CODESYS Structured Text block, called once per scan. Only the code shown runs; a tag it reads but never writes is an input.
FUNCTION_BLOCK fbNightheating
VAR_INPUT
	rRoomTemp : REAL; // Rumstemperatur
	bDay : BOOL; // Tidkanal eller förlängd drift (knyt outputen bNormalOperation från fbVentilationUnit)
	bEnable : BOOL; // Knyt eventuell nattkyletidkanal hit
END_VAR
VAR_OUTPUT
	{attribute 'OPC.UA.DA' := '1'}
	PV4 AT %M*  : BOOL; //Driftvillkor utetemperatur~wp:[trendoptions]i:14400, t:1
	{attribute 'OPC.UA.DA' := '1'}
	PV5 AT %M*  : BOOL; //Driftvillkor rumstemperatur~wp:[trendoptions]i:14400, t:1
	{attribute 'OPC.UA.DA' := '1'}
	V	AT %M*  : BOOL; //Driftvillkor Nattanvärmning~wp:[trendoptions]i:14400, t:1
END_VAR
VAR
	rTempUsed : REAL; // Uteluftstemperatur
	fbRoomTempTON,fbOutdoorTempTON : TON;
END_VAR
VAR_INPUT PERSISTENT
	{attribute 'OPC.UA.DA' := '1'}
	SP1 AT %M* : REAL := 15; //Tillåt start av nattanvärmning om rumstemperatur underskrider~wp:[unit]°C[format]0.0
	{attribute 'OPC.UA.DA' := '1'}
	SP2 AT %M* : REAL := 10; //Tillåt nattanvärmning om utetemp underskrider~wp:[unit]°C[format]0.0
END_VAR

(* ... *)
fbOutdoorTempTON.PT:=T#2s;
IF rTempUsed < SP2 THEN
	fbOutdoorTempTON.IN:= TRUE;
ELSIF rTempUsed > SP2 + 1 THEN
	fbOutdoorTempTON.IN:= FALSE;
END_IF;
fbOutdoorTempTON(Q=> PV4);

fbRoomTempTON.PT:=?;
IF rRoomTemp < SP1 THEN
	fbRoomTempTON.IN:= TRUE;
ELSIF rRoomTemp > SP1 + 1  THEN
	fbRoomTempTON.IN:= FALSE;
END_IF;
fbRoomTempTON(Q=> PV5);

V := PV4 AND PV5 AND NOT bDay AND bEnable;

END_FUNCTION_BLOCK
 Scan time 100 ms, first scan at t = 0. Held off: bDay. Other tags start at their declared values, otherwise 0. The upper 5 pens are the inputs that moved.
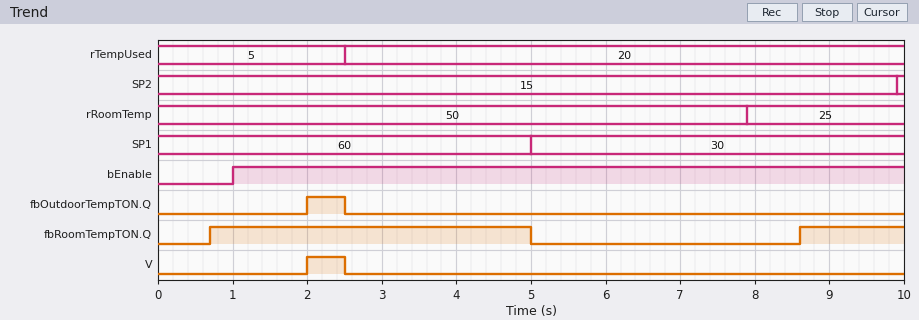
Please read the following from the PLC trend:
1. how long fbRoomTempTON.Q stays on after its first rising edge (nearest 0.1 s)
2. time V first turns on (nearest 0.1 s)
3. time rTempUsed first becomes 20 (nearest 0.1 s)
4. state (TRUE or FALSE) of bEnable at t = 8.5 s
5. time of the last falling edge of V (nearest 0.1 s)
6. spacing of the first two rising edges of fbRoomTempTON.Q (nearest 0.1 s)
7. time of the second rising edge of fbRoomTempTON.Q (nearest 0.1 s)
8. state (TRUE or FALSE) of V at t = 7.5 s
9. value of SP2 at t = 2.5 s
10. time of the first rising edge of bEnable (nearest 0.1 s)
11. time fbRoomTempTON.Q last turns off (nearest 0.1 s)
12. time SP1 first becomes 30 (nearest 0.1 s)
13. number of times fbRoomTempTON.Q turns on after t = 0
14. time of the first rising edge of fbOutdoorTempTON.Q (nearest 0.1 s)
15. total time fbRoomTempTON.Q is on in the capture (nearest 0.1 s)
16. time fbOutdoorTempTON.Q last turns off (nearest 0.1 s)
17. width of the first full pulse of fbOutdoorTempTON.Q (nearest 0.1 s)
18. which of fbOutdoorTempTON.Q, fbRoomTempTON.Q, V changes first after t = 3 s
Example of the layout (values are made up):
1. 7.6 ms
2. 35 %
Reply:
1. 4.3 s
2. 2.0 s
3. 2.5 s
4. TRUE
5. 2.5 s
6. 7.9 s
7. 8.6 s
8. FALSE
9. 15
10. 1.0 s
11. 5.0 s
12. 5.0 s
13. 2
14. 2.0 s
15. 5.7 s
16. 2.5 s
17. 0.5 s
18. fbRoomTempTON.Q
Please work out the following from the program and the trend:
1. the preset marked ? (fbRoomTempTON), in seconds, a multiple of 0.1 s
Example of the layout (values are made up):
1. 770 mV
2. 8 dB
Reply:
1. 0.7 s
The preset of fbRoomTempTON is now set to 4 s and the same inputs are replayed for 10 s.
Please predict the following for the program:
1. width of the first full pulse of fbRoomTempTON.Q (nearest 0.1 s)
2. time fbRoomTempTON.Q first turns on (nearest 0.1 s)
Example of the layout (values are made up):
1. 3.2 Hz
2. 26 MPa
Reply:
1. 1.0 s
2. 4.0 s
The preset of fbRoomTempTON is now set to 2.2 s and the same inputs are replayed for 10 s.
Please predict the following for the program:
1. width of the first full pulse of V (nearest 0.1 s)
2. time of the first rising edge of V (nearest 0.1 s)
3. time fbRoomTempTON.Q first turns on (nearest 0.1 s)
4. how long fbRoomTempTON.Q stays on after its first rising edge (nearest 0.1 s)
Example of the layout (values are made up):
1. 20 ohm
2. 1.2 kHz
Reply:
1. 0.3 s
2. 2.2 s
3. 2.2 s
4. 2.8 s
